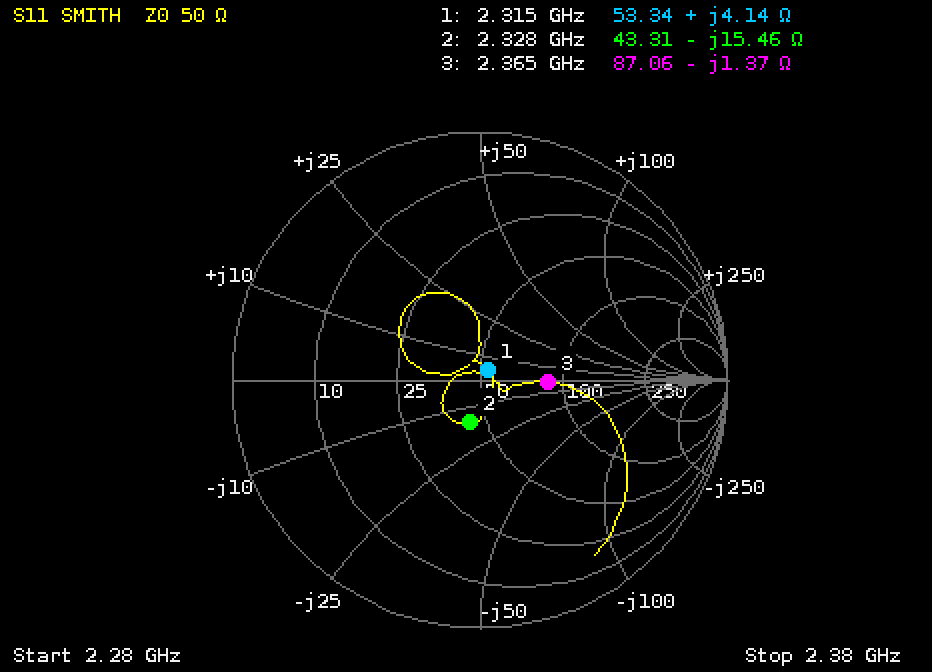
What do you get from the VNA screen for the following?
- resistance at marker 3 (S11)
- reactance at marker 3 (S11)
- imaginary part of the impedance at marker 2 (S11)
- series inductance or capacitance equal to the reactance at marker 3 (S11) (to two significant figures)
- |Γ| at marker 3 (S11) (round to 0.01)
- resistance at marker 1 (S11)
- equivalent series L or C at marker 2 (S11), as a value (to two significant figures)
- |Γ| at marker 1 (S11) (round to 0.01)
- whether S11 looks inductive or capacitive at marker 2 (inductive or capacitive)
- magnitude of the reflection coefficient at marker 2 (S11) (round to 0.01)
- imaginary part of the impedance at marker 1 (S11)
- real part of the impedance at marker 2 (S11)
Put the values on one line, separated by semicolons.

87.06 Ω; -1.37 Ω; -15.46 Ω; 49 pF; 0.27; 53.34 Ω; 4.4 pF; 0.05; capacitive; 0.18; +4.14 Ω; 43.31 Ω
